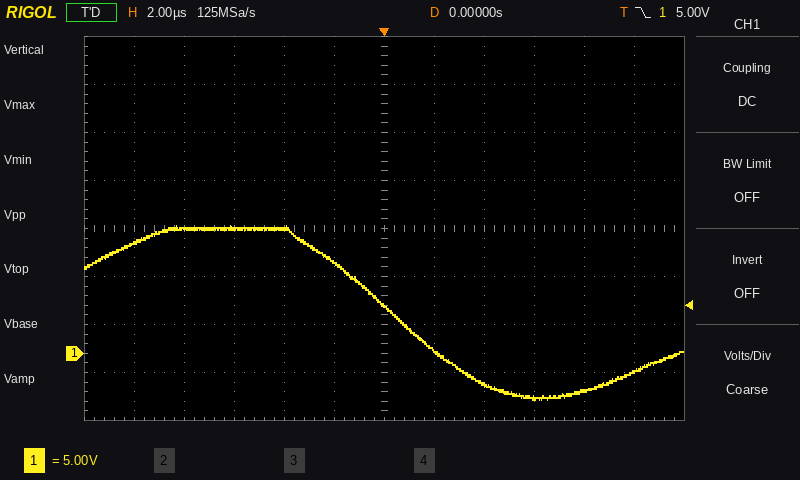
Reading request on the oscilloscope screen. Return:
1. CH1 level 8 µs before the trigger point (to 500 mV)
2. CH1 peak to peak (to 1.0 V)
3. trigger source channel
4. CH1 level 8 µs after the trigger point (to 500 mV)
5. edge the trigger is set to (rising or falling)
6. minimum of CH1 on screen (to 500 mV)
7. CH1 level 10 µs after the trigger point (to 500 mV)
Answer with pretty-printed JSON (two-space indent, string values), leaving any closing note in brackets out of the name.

{
  "CH1 level 8 µs before the trigger point": "13.0 V",
  "CH1 peak to peak": "18.0 V",
  "trigger source channel": "CH1",
  "CH1 level 8 µs after the trigger point": "-4.0 V",
  "edge the trigger is set to": "falling",
  "minimum of CH1 on screen": "-5.0 V",
  "CH1 level 10 µs after the trigger point": "-2.0 V"
}
